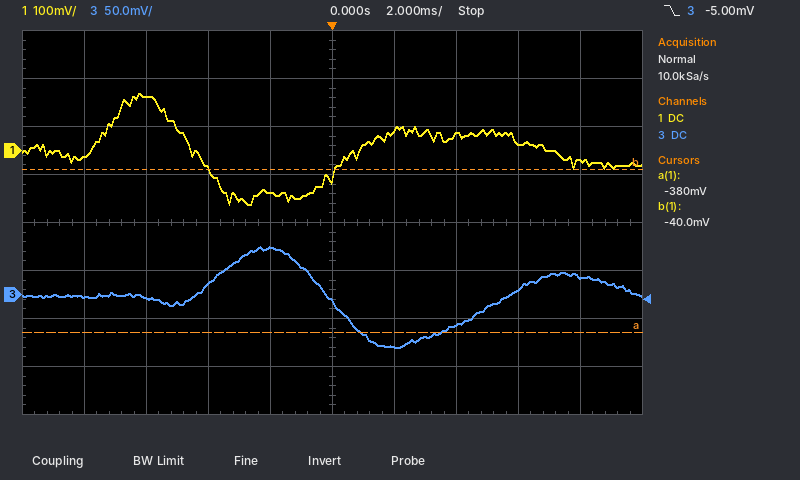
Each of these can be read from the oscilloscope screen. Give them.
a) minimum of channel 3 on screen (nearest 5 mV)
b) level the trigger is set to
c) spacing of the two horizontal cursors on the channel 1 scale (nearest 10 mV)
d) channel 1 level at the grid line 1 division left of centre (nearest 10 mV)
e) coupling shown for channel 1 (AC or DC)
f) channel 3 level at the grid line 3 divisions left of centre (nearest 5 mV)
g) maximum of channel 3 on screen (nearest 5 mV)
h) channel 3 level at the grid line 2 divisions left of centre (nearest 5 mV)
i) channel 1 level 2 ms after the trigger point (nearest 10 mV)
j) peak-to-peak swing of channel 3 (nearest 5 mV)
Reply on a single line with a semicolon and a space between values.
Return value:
-55 mV; -5.00 mV; 340 mV; -90 mV; DC; -5 mV; 50 mV; 10 mV; 40 mV; 105 mV
